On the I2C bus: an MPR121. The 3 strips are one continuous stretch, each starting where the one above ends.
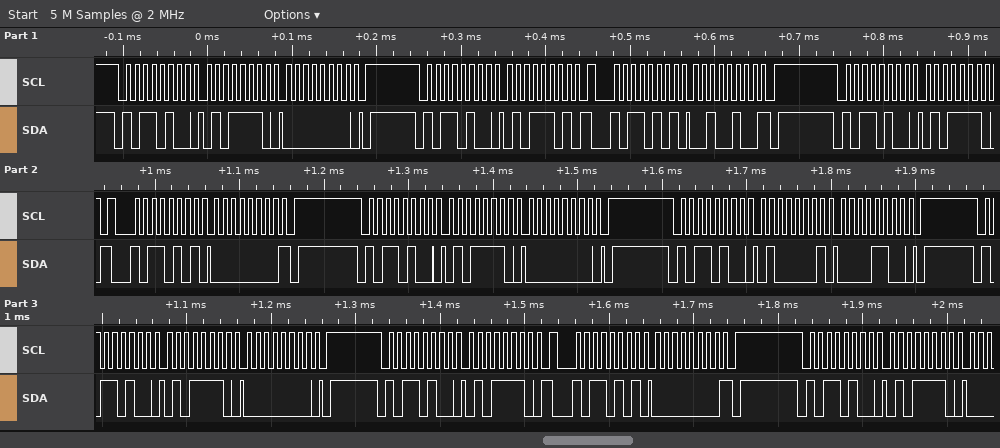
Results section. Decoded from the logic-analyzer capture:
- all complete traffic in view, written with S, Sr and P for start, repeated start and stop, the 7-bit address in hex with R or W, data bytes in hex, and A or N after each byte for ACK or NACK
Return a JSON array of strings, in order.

["S 5AW A 5E A 00 A P S 5AW A 5D A Sr 5AR A 24 N P S 5AW A 5E A Sr 5AR A 00 N P S 5AW A 5E A 00 A P S 5AW A 41 A 0C A P S 5AW A 5E A 00 A P S 5AW A 5E A Sr 5AR A 00 N P S 5AW A 5E A"]
